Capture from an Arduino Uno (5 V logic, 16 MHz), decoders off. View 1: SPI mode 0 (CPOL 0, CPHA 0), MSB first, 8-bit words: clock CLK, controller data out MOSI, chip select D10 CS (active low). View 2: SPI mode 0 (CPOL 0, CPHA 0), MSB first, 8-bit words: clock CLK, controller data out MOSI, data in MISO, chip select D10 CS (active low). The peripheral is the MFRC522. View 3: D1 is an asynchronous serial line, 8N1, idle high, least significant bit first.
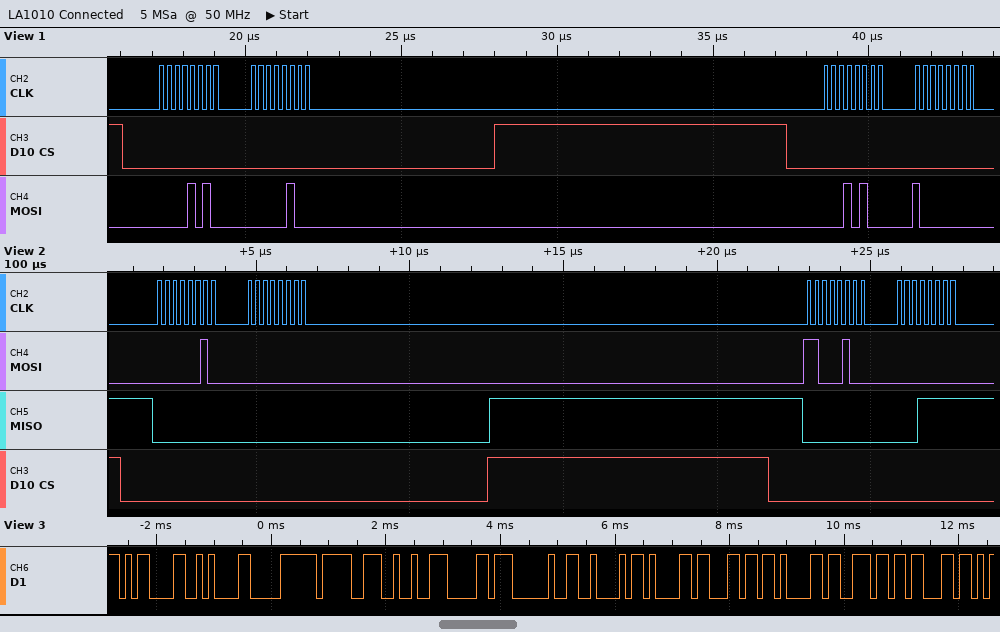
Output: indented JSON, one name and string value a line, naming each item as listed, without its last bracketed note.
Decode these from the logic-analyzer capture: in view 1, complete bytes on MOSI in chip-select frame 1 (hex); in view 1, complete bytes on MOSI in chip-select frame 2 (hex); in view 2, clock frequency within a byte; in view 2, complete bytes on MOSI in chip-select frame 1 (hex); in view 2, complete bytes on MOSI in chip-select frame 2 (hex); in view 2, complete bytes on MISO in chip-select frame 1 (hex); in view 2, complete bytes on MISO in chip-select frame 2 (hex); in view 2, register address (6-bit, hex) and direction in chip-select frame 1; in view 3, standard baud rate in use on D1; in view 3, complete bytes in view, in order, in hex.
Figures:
{
  "in view 1, complete bytes on MOSI in chip-select frame 1": "0x0A 0x04",
  "in view 1, complete bytes on MOSI in chip-select frame 2": "0x14 0x80",
  "in view 2, clock frequency within a byte": "4 MHz",
  "in view 2, complete bytes on MOSI in chip-select frame 1": "02 00",
  "in view 2, complete bytes on MOSI in chip-select frame 2": "C4 00",
  "in view 2, complete bytes on MISO in chip-select frame 1": "00 00",
  "in view 2, complete bytes on MISO in chip-select frame 2": "00 1F",
  "in view 2, register address (6-bit, hex) and direction in chip-select frame 1": "0x01 write",
  "in view 3, standard baud rate in use on D1": "9600 baud",
  "in view 3, complete bytes in view, in order, in hex": "0D 0A F0 9F 92 B0 20 42 61 6C 61 6E 63"
}
